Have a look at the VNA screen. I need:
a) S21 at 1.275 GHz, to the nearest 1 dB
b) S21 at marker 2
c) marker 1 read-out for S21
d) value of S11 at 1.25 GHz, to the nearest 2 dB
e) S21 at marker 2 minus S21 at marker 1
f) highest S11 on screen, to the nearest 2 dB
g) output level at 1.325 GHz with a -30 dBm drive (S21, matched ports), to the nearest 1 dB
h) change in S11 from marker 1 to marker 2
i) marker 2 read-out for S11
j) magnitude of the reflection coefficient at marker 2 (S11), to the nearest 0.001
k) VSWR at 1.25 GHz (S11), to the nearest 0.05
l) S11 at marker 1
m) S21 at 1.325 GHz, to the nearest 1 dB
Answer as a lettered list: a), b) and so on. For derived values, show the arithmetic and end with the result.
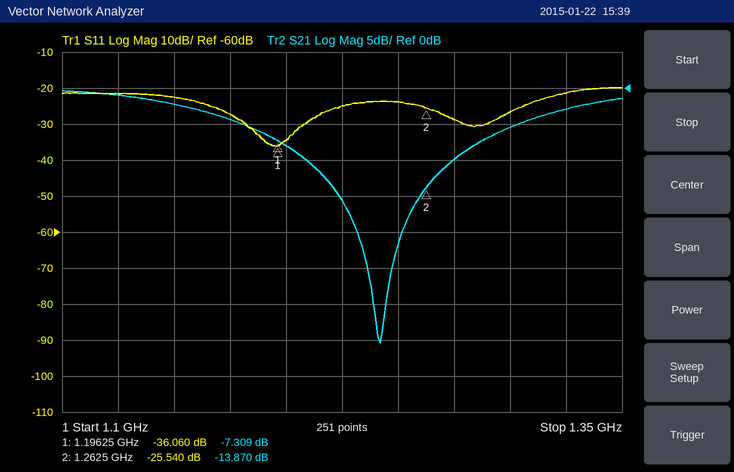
a) -10 dB
b) -13.870 dB
c) -7.309 dB
d) -24 dB
e) -13.87 − (-7.309) = -6.561 dB
f) -20 dB
g) -30 dBm + (-3 dB) = -33 dBm
h) -25.54 − (-36.06) = 10.520 dB
i) -25.540 dB
j) 10^(-25.54/20) ≈ 0.053
k) |Γ| = 10^(-24/20) = 0.0631; VSWR = (1 + 0.0631)/(1 − 0.0631) ≈ 1.13, so 1.15 to the nearest 0.05
l) -36.060 dB
m) -3 dB
